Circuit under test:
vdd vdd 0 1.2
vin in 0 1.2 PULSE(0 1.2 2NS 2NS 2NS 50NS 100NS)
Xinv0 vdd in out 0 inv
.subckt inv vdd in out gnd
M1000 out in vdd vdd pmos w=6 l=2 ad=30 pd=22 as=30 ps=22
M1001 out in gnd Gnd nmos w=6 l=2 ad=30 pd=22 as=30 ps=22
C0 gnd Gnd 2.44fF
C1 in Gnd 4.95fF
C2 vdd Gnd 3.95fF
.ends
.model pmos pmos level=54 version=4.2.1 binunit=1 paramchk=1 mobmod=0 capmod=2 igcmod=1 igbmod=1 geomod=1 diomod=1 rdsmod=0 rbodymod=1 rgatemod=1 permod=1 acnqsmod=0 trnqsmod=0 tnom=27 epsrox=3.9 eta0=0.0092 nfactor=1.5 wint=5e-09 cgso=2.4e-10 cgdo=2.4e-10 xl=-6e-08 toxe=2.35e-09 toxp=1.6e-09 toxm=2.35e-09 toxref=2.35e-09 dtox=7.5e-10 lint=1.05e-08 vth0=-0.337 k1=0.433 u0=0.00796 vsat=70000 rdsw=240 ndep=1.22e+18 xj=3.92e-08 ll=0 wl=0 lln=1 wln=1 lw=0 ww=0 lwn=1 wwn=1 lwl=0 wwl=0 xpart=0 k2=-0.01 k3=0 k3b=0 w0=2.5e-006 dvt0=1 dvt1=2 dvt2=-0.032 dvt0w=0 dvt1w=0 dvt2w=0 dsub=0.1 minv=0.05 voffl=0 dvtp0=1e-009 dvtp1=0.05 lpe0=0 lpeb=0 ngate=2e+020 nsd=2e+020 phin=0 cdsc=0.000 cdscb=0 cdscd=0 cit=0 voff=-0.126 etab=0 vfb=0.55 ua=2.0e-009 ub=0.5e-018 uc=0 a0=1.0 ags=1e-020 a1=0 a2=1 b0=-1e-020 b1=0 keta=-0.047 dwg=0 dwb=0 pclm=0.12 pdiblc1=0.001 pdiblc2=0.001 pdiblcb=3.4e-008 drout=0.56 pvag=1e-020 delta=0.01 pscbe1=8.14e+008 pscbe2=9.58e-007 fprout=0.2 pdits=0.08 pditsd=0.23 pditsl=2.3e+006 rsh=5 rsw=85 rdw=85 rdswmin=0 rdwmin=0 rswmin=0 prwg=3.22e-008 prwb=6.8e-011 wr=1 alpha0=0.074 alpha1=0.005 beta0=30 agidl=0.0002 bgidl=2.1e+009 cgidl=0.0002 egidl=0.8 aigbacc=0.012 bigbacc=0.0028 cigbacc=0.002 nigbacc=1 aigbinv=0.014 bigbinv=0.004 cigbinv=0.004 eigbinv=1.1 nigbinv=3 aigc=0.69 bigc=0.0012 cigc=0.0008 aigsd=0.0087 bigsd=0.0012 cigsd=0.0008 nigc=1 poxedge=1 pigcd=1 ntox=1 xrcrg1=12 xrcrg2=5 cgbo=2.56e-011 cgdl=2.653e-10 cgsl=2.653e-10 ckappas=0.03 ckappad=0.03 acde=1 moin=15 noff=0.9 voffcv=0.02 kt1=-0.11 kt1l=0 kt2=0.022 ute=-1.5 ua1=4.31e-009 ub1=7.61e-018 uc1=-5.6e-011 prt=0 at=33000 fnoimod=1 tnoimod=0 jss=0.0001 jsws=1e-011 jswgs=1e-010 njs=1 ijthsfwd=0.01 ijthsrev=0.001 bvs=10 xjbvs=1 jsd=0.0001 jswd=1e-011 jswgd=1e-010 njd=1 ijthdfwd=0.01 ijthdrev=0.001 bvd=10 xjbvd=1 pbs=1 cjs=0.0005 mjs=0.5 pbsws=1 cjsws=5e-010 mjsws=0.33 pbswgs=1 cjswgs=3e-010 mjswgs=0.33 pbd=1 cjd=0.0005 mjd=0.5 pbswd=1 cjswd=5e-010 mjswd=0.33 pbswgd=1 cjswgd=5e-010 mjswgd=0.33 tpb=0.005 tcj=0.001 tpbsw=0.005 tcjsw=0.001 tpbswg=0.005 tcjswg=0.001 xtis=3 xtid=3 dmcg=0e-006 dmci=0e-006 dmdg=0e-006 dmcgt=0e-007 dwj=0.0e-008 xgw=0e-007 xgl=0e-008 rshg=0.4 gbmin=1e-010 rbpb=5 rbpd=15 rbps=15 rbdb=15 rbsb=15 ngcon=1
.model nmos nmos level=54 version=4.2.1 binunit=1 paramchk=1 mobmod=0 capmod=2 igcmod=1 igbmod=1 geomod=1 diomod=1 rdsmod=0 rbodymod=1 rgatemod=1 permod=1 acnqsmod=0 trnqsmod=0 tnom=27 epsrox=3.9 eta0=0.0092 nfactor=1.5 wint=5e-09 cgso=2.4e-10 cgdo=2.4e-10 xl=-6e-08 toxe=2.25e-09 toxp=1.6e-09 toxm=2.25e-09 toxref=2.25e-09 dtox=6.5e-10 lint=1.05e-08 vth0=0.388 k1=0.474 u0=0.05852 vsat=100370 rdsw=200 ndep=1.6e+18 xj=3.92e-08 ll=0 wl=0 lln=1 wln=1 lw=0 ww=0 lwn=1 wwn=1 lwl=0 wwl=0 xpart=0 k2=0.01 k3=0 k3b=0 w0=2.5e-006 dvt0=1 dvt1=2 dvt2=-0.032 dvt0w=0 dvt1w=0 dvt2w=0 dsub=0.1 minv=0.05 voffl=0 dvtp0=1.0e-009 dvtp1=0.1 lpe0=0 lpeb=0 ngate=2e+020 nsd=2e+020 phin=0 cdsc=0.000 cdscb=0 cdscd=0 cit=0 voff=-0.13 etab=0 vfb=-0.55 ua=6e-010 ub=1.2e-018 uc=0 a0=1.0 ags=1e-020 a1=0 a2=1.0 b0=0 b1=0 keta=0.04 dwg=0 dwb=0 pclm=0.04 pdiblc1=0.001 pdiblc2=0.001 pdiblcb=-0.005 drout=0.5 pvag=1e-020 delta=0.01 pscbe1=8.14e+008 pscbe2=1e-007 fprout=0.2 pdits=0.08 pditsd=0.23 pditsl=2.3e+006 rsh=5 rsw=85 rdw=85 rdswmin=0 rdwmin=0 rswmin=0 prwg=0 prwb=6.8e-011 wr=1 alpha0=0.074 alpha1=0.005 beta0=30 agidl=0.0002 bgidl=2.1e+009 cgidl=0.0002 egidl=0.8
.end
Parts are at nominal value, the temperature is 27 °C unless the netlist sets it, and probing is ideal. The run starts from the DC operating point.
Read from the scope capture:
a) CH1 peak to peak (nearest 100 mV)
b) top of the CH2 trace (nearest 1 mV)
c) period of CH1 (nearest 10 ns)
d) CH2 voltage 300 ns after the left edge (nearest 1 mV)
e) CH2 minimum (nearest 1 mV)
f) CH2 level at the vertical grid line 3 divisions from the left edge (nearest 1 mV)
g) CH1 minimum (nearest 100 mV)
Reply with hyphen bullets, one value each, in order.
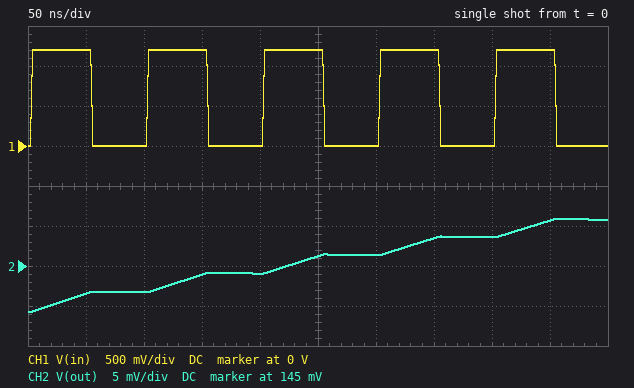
- 1.2 V
- 151 mV
- 100 ns
- 146 mV
- 139 mV
- 144 mV
- 0 V
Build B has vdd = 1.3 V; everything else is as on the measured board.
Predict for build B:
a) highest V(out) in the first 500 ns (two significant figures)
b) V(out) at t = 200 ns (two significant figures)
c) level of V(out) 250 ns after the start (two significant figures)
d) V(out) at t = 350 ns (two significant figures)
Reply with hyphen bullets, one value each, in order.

- 18 mV
- 2.1 mV
- 7.5 mV
- 13 mV
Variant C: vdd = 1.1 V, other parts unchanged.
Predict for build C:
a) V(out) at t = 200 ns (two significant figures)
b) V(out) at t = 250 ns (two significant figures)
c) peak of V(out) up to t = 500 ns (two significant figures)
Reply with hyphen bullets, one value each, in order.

- 150 mV
- 150 mV
- 160 mV
